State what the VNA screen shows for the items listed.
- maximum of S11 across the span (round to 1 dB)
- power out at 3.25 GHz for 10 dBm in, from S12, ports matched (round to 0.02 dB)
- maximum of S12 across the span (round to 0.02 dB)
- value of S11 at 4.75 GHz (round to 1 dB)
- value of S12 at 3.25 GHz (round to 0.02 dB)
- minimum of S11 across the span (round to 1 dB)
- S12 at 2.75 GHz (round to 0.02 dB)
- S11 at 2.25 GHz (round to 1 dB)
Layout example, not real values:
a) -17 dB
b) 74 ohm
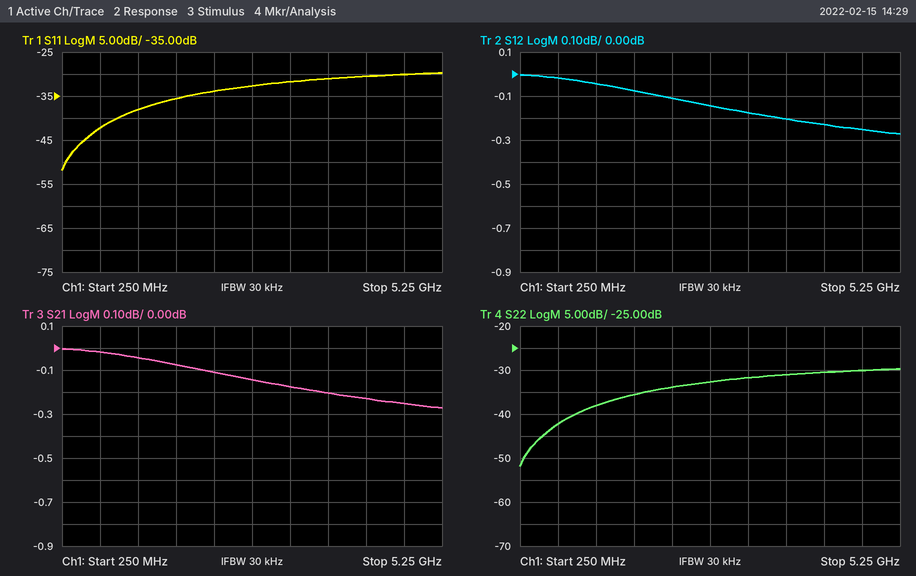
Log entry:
a) -30 dB
b) 9.82 dBm
c) 0.00 dB
d) -30 dB
e) -0.18 dB
f) -52 dB
g) -0.14 dB
h) -34 dB
